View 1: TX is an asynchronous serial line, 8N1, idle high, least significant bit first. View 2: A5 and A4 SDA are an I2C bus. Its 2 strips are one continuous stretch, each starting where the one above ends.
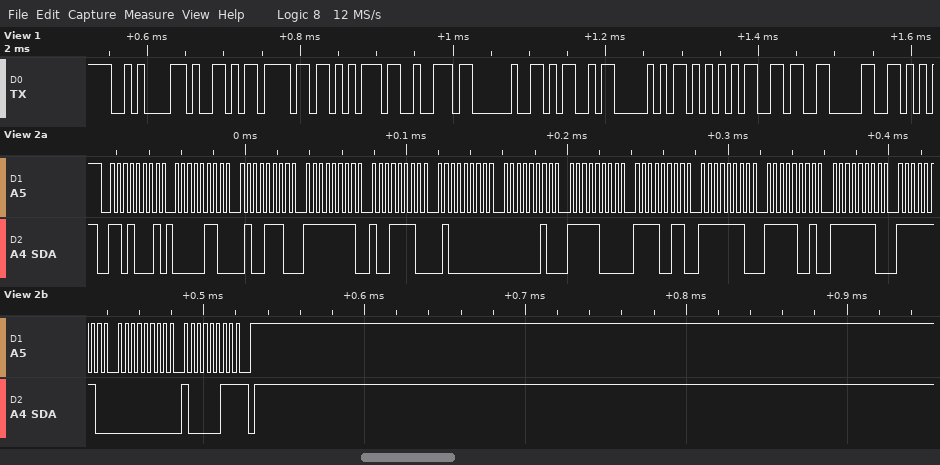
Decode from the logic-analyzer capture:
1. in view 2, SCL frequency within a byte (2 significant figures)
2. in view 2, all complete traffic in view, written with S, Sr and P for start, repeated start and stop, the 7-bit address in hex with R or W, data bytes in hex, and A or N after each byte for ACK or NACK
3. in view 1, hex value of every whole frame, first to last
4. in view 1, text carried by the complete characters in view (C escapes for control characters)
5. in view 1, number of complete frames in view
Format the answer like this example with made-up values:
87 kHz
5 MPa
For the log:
250 kHz
S 68R A 06 A 4E A FF A 9E A 40 A 02 A F8 A F3 A FE A F9 A FE A FE A 00 A 83 N P
0A 59 6F 75 72 20 4D 50 55 36 30
"\nYour MPU60"
11
